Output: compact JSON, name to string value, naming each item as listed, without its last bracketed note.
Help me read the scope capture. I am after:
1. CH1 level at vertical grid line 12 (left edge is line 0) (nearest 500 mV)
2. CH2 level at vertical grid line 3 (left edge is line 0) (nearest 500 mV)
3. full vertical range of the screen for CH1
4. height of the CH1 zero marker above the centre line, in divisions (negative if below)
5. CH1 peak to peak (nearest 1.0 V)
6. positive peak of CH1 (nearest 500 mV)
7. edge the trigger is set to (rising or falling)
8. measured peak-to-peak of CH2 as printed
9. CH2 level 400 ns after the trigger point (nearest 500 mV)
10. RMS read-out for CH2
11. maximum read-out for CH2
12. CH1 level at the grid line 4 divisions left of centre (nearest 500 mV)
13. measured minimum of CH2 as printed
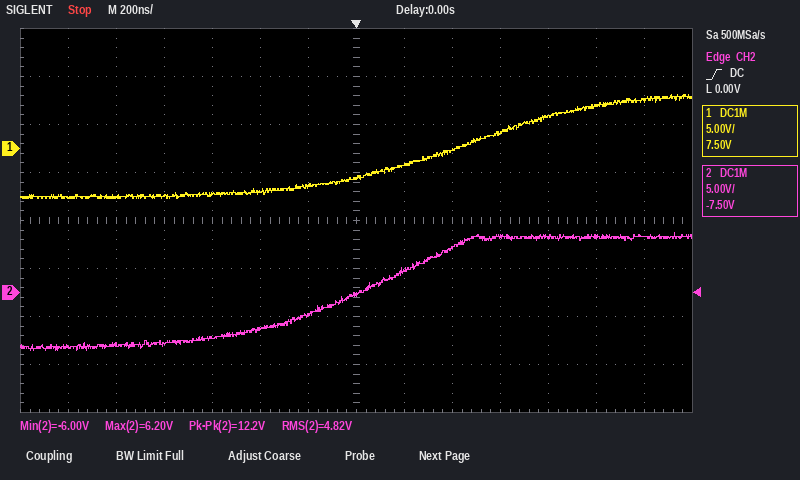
{"CH1 level at vertical grid line 12 (left edge is line 0)": "4.5 V", "CH2 level at vertical grid line 3 (left edge is line 0)": "-5.5 V", "full vertical range of the screen for CH1": "40 V", "height of the CH1 zero marker above the centre line, in divisions": "+1.5 div", "CH1 peak to peak": "11.0 V", "positive peak of CH1": "5.5 V", "edge the trigger is set to": "rising", "measured peak-to-peak of CH2 as printed": "12.2 V", "CH2 level 400 ns after the trigger point": "4.5 V", "RMS read-out for CH2": "4.82 V", "maximum read-out for CH2": "6.20 V", "CH1 level at the grid line 4 divisions left of centre": "-5.0 V", "measured minimum of CH2 as printed": "-6.00 V"}
